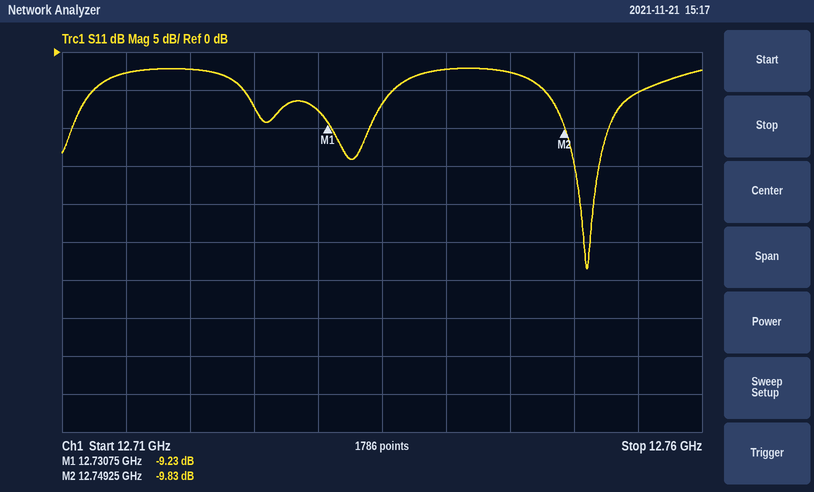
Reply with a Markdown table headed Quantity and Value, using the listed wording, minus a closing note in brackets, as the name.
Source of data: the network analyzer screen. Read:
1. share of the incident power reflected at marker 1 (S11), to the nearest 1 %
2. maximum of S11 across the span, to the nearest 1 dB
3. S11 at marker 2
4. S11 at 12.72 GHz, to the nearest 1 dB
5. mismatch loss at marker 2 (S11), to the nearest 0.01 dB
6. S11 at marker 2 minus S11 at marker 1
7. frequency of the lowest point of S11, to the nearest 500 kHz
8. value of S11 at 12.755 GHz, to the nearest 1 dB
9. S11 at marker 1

| Quantity | Value |
|---|---|
| share of the incident power reflected at marker 1 (S11), to the nearest 1 % | 12 % |
| maximum of S11 across the span, to the nearest 1 dB | -2 dB |
| S11 at marker 2 | -9.83 dB |
| S11 at 12.72 GHz, to the nearest 1 dB | -2 dB |
| mismatch loss at marker 2 (S11), to the nearest 0.01 dB | 0.48 dB |
| S11 at marker 2 minus S11 at marker 1 | -0.60 dB |
| frequency of the lowest point of S11, to the nearest 500 kHz | 12.7510 GHz |
| value of S11 at 12.755 GHz, to the nearest 1 dB | -5 dB |
| S11 at marker 1 | -9.23 dB |
